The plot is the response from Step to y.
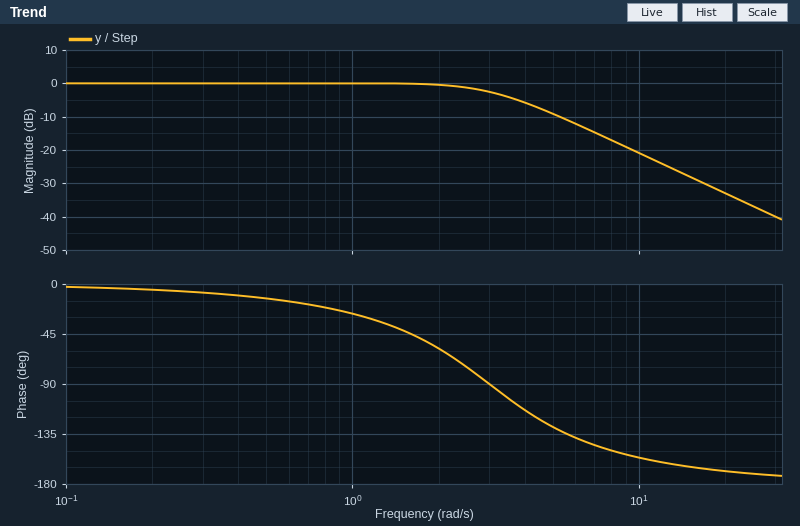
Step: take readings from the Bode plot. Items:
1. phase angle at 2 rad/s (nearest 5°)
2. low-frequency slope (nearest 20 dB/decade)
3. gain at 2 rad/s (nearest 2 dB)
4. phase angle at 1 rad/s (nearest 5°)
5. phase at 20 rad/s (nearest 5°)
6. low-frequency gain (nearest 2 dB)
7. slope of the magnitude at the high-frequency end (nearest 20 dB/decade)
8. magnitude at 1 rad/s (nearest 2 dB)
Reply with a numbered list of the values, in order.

1. -60°
2. 0 dB/decade
3. 0 dB
4. -25°
5. -170°
6. 0 dB
7. -40 dB/decade
8. 0 dB
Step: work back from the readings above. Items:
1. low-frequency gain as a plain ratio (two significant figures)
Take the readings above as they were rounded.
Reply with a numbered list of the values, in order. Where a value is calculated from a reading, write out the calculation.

1. 10^(0 / 20) = 1.0
